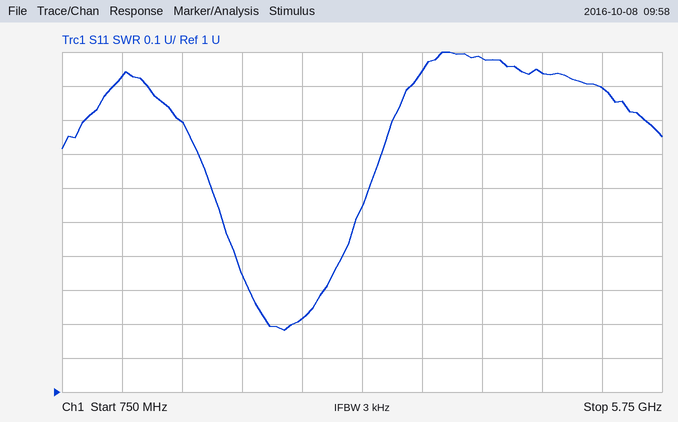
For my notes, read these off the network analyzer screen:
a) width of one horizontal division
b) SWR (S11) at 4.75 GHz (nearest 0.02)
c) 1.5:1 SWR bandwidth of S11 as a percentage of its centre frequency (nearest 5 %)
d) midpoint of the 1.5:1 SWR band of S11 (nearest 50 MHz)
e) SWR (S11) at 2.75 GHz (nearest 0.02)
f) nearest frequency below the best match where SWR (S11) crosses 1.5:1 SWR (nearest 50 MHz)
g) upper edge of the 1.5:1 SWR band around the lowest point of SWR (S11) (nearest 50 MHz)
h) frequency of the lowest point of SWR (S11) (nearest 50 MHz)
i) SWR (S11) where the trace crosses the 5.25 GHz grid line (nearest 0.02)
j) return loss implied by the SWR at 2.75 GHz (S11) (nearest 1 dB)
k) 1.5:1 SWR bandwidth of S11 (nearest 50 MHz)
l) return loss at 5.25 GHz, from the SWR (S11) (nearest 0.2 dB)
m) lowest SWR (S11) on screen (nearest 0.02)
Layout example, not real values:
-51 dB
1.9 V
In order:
500 MHz
1.94
40 %
2.65 GHz
1.22
2.10 GHz
3.20 GHz
2.60 GHz
1.90
20 dB
1.10 GHz
10.2 dB
1.18
